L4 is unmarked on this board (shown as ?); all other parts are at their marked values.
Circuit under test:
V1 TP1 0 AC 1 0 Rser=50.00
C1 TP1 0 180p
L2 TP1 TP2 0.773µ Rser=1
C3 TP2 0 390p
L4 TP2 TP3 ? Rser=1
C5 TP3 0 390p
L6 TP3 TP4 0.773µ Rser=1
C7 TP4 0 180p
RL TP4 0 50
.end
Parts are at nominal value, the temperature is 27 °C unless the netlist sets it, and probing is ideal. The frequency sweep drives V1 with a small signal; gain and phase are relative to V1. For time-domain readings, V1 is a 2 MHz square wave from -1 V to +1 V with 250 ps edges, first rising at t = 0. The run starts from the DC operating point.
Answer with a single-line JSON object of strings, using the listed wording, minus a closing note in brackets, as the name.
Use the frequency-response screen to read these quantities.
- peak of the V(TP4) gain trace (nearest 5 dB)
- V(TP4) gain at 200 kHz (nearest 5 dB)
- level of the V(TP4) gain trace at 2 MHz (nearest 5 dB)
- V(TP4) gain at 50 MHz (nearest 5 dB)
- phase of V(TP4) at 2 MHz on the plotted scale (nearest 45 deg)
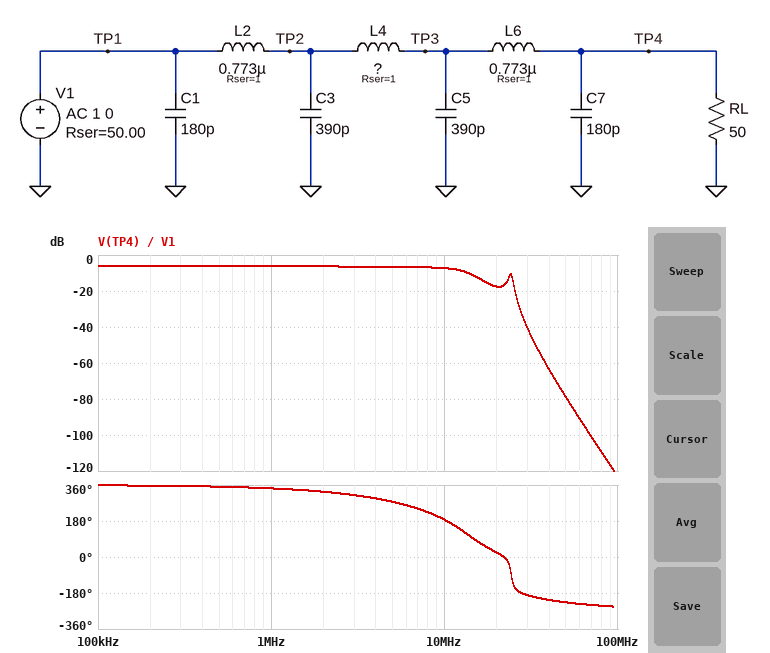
{"peak of the V(TP4) gain trace": "-5 dB", "V(TP4) gain at 200 kHz": "-5 dB", "level of the V(TP4) gain trace at 2 MHz": "-5 dB", "V(TP4) gain at 50 MHz": "-80 dB", "phase of V(TP4) at 2 MHz on the plotted scale": "315 deg"}
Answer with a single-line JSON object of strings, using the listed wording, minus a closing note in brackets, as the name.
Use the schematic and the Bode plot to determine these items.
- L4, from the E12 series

{"L4, from the E12 series": "270 nH"}
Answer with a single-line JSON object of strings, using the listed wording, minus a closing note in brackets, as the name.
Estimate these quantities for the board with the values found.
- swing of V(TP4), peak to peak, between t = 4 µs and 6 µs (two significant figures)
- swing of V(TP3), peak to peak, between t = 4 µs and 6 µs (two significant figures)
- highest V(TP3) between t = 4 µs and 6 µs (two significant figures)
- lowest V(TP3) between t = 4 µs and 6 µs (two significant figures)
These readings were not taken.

{"swing of V(TP4), peak to peak, between t = 4 µs and 6 µs": "1.1 V", "swing of V(TP3), peak to peak, between t = 4 µs and 6 µs": "1.1 V", "highest V(TP3) between t = 4 µs and 6 µs": "550 mV", "lowest V(TP3) between t = 4 µs and 6 µs": "-550 mV"}
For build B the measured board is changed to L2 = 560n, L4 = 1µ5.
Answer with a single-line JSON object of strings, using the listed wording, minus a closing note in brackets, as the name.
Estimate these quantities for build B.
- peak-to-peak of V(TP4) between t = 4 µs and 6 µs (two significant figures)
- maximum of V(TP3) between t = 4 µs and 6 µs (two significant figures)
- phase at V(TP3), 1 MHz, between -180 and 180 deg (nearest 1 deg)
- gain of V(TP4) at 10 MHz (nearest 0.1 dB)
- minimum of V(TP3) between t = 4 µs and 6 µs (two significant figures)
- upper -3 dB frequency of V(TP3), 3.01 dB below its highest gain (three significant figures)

{"peak-to-peak of V(TP4) between t = 4 µs and 6 µs": "1.2 V", "maximum of V(TP3) between t = 4 µs and 6 µs": "590 mV", "phase at V(TP3), 1 MHz, between -180 and 180 deg": "-15 deg", "gain of V(TP4) at 10 MHz": "-8.1 dB", "minimum of V(TP3) between t = 4 µs and 6 µs": "-590 mV", "upper -3 dB frequency of V(TP3), 3.01 dB below its highest gain": "14.8 MHz"}
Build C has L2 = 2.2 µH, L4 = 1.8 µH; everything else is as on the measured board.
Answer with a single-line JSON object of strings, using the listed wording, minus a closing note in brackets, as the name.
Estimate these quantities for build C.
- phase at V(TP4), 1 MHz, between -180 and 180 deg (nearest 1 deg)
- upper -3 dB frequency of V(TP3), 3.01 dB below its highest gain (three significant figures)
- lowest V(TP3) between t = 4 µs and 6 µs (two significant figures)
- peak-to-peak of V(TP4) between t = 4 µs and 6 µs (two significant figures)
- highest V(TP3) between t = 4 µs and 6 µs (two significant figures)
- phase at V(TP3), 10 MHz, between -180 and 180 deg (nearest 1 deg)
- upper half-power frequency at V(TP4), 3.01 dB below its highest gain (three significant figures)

{"phase at V(TP4), 1 MHz, between -180 and 180 deg": "-27 deg", "upper -3 dB frequency of V(TP3), 3.01 dB below its highest gain": "10.0 MHz", "lowest V(TP3) between t = 4 µs and 6 µs": "-580 mV", "peak-to-peak of V(TP4) between t = 4 µs and 6 µs": "1.2 V", "highest V(TP3) between t = 4 µs and 6 µs": "580 mV", "phase at V(TP3), 10 MHz, between -180 and 180 deg": "112 deg", "upper half-power frequency at V(TP4), 3.01 dB below its highest gain": "9.84 MHz"}
